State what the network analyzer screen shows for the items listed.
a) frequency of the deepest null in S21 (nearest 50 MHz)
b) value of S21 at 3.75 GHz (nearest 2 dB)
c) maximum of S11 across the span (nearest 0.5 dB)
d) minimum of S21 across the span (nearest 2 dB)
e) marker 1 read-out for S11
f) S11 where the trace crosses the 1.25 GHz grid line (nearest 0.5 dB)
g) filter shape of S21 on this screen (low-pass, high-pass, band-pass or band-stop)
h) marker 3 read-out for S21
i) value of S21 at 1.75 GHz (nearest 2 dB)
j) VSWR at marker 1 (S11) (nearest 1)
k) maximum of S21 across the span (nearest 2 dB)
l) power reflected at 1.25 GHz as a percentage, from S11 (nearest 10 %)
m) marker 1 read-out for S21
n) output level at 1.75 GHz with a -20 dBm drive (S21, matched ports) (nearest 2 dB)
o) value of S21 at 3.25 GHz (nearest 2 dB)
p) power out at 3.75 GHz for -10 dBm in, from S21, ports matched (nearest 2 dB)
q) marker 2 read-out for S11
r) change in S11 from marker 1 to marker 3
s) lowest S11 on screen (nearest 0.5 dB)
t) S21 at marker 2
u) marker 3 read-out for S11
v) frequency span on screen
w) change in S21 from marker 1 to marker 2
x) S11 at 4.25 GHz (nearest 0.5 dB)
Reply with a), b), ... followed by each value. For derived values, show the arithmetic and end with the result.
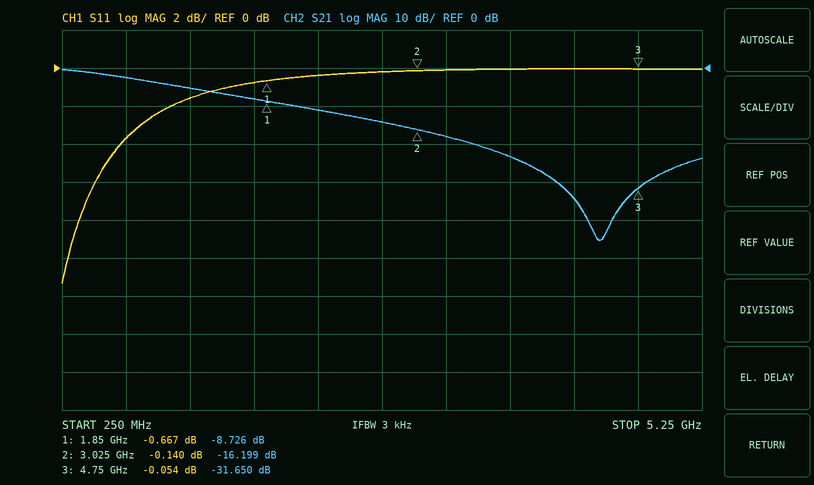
a) 4.45 GHz
b) -24 dB
c) 0.0 dB
d) -46 dB
e) -0.667 dB
f) -1.5 dB
g) low-pass
h) -31.650 dB
i) -8 dB
j) (1 + 0.9261)/(1 − 0.9261) ≈ 26
k) 0 dB
l) 10^(-1.5/10) ≈ 70.8 %, so 70 % to the nearest 10 %
m) -8.726 dB
n) -20 dBm + (-8 dB) = -28 dBm
o) -18 dB
p) -10 dBm + (-24 dB) = -34 dBm
q) -0.140 dB
r) -0.054 − (-0.667) = 0.613 dB
s) -11.5 dB
t) -16.199 dB
u) -0.054 dB
v) 5 GHz
w) -16.199 − (-8.726) = -7.473 dB
x) 0.0 dB
